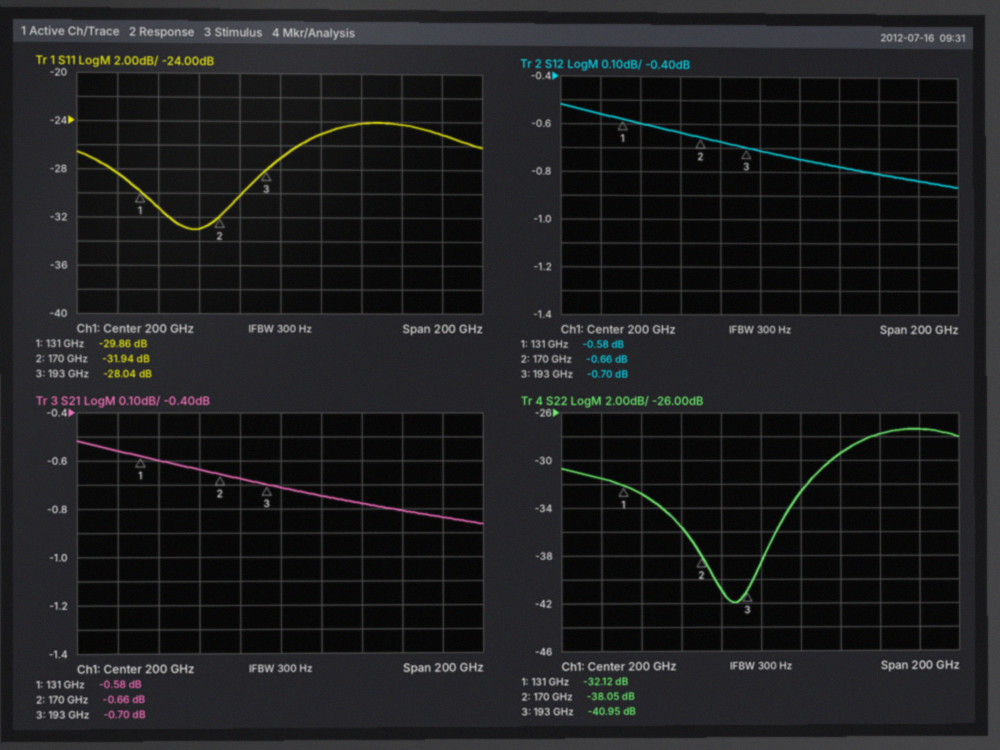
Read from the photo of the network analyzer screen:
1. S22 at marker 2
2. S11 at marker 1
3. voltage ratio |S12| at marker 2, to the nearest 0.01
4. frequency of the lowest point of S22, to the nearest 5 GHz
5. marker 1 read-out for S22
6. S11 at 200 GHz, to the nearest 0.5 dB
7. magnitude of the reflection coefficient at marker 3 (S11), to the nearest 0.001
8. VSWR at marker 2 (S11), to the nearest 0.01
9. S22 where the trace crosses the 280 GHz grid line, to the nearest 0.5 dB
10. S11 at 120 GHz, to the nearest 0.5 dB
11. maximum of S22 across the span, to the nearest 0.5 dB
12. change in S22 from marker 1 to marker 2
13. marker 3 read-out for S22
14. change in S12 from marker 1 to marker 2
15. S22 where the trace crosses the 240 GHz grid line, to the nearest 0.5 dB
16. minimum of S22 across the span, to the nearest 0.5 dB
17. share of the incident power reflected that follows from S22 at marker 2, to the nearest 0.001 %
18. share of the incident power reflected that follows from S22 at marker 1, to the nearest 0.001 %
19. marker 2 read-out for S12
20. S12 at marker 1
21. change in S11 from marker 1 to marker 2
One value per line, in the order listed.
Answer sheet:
-38.05 dB
-29.86 dB
0.93
185 GHz
-32.12 dB
-27.0 dB
0.040
1.05
-27.5 dB
-28.5 dB
-27.5 dB
-5.93 dB
-40.95 dB
-0.08 dB
-29.5 dB
-42.0 dB
0.016 %
0.061 %
-0.66 dB
-0.58 dB
-2.08 dB
